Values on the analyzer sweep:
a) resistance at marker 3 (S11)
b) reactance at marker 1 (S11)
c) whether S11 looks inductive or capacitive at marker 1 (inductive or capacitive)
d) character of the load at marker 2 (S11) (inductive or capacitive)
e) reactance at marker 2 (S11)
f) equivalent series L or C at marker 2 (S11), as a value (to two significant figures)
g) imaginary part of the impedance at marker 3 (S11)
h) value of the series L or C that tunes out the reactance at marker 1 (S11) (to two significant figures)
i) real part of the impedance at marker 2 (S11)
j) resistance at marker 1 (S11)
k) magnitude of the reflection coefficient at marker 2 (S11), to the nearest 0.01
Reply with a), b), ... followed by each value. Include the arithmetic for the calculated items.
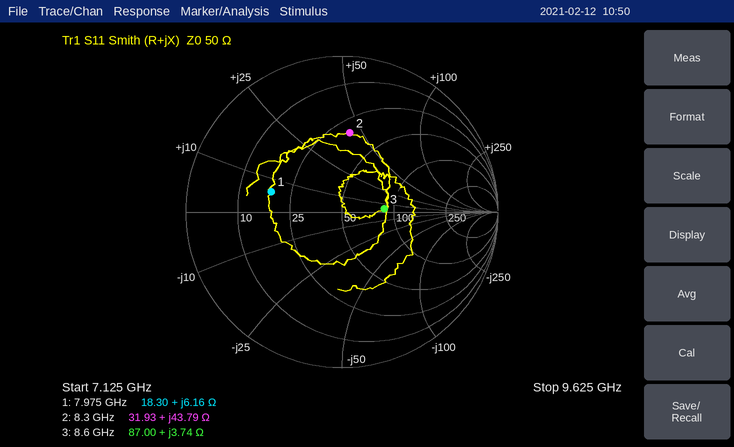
a) 87.00 Ω
b) +6.16 Ω
c) inductive
d) inductive
e) +43.79 Ω
f) L = 43.79 Ω/(2π × 8.3 GHz) ≈ 840 pH
g) +3.74 Ω
h) C = 1/(2π × 7.975 GHz × 6.16 Ω) ≈ 3.2 pF
i) 31.93 Ω
j) 18.30 Ω
k) 0.51
